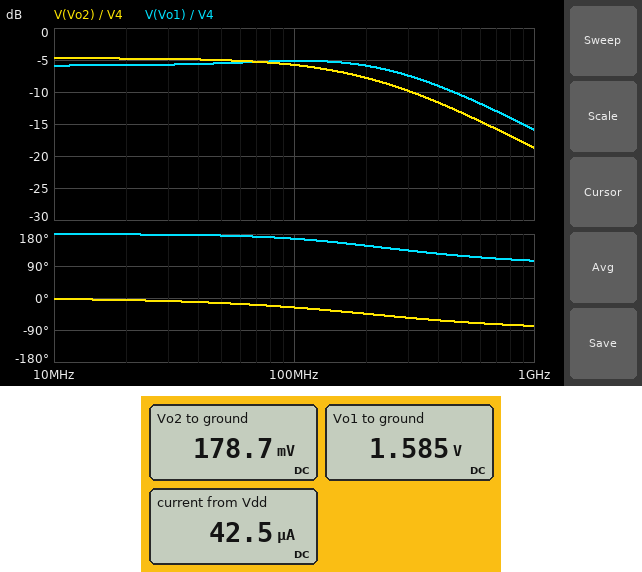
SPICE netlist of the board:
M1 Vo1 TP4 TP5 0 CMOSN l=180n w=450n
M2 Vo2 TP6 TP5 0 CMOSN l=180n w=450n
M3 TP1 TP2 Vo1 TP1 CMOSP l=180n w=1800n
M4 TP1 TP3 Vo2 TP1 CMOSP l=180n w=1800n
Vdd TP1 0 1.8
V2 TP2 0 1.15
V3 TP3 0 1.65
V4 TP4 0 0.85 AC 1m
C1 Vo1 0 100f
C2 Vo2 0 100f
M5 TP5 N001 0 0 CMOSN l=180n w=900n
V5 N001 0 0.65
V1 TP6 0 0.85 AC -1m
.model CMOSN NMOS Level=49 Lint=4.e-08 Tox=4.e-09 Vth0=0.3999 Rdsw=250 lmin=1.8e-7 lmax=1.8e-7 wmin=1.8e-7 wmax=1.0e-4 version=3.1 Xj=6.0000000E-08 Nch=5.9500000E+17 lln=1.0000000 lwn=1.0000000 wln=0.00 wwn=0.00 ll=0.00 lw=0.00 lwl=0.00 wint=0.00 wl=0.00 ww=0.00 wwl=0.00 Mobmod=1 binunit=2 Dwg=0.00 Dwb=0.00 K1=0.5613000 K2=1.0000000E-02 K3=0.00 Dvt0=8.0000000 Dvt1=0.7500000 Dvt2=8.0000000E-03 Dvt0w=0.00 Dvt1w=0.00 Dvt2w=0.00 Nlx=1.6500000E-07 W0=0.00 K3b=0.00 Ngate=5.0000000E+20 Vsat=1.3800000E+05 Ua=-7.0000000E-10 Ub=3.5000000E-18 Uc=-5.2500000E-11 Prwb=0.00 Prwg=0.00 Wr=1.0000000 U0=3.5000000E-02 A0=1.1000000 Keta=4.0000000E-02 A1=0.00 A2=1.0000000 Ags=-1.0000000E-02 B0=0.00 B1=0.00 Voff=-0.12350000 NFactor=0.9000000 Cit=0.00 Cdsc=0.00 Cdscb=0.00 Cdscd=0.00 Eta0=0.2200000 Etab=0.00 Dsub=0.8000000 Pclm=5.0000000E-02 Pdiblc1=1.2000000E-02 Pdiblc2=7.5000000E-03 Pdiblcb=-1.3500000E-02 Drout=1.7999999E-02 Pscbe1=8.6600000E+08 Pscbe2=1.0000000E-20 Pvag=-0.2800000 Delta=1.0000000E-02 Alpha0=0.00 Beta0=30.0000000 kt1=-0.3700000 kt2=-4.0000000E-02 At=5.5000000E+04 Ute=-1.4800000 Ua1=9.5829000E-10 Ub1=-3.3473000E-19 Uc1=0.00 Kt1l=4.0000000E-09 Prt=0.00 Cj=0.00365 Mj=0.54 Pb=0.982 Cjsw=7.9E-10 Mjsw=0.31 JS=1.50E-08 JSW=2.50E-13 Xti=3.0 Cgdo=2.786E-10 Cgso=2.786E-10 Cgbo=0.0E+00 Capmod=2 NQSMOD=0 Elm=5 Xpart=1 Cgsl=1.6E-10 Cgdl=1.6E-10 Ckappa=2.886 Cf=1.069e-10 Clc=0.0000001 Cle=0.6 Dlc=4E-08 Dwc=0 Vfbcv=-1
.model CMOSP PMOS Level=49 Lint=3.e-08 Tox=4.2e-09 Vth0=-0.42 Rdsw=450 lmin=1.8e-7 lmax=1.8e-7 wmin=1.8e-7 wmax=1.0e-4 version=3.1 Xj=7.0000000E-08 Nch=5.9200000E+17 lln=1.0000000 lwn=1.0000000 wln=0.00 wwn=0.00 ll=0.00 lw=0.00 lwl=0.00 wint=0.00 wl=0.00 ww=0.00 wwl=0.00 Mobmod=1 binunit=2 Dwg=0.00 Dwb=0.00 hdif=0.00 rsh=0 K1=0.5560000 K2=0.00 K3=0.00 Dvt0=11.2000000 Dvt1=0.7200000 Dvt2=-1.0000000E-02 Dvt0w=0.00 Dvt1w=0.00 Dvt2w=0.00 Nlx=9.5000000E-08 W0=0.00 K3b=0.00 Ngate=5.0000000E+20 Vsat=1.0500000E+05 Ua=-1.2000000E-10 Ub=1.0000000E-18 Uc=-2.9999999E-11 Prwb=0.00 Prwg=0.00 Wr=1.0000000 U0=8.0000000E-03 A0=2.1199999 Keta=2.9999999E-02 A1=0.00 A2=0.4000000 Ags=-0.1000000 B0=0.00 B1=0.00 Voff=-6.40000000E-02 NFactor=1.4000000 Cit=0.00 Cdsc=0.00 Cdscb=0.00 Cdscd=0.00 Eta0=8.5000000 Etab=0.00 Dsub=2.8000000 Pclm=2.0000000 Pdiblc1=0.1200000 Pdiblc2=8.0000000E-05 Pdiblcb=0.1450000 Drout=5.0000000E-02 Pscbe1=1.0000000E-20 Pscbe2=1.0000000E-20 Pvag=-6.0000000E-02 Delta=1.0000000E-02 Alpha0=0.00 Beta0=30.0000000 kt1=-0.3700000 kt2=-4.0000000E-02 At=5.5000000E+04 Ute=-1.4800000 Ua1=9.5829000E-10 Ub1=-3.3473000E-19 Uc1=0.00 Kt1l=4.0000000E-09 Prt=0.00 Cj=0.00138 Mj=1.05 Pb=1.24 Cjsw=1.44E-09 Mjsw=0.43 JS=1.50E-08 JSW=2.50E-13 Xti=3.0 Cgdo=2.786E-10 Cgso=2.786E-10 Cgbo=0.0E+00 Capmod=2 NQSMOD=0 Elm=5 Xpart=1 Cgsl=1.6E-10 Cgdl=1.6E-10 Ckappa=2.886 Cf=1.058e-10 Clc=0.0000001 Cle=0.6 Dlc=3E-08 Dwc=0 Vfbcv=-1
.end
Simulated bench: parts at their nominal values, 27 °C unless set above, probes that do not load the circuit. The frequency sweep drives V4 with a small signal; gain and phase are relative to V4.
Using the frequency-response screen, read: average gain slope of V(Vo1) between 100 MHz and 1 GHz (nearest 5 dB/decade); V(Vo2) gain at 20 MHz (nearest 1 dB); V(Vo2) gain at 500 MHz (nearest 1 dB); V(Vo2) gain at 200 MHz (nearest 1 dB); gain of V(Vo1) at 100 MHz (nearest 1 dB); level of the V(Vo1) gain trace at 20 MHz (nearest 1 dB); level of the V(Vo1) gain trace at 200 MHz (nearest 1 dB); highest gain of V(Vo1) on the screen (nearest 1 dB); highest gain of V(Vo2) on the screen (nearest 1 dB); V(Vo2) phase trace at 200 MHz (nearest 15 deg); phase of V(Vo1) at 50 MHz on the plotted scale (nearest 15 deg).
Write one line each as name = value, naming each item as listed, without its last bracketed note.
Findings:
average gain slope of V(Vo1) between 100 MHz and 1 GHz = -10 dB/decade
V(Vo2) gain at 20 MHz = -5 dB
V(Vo2) gain at 500 MHz = -13 dB
V(Vo2) gain at 200 MHz = -8 dB
gain of V(Vo1) at 100 MHz = -5 dB
level of the V(Vo1) gain trace at 20 MHz = -6 dB
level of the V(Vo1) gain trace at 200 MHz = -6 dB
highest gain of V(Vo1) on the screen = -5 dB
highest gain of V(Vo2) on the screen = -5 dB
V(Vo2) phase trace at 200 MHz = -45 deg
phase of V(Vo1) at 50 MHz on the plotted scale = 180 deg
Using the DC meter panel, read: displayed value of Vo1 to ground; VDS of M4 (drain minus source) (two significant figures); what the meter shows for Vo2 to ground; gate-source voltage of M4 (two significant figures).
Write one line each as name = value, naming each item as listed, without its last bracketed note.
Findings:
displayed value of Vo1 to ground = 1.585 V
VDS of M4 (drain minus source) = 1.6 V
what the meter shows for Vo2 to ground = 178.7 mV
gate-source voltage of M4 = 1.5 V
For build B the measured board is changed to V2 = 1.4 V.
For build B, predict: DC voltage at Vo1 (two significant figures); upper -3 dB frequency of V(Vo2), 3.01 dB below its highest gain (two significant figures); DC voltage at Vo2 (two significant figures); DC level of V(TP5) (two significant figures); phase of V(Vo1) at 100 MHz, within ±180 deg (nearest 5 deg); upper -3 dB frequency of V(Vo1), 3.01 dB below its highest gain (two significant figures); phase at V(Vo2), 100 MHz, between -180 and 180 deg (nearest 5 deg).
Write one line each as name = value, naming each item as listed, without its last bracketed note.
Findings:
DC voltage at Vo1 = 96 mV
upper -3 dB frequency of V(Vo2), 3.01 dB below its highest gain = 720 MHz
DC voltage at Vo2 = 43 mV
DC level of V(TP5) = 42 mV
phase of V(Vo1) at 100 MHz, within ±180 deg = 155 deg
upper -3 dB frequency of V(Vo1), 3.01 dB below its highest gain = 210 MHz
phase at V(Vo2), 100 MHz, between -180 and 180 deg = 40 deg
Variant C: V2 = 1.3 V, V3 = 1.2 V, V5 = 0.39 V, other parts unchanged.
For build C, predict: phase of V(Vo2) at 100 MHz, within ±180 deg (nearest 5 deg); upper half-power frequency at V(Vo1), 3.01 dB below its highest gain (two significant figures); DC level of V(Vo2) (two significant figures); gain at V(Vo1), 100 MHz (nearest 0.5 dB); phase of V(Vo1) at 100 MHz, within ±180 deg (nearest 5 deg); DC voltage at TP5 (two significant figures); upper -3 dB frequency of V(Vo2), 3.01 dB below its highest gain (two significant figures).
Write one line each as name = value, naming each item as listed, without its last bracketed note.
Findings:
phase of V(Vo2) at 100 MHz, within ±180 deg = -15 deg
upper half-power frequency at V(Vo1), 3.01 dB below its highest gain = 250 MHz
DC level of V(Vo2) = 1.8 V
gain at V(Vo1), 100 MHz = -23.5 dB
phase of V(Vo1) at 100 MHz, within ±180 deg = 160 deg
DC voltage at TP5 = 460 mV
upper -3 dB frequency of V(Vo2), 3.01 dB below its highest gain = 380 MHz
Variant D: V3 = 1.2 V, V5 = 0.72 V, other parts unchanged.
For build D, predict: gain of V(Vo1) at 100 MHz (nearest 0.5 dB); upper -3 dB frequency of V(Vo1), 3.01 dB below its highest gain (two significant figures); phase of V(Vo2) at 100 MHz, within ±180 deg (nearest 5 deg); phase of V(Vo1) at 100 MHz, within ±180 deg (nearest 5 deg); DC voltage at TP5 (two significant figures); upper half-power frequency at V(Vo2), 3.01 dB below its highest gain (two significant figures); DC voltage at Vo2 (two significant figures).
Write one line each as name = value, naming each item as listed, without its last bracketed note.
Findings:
gain of V(Vo1) at 100 MHz = -4.5 dB
upper -3 dB frequency of V(Vo1), 3.01 dB below its highest gain = 270 MHz
phase of V(Vo2) at 100 MHz, within ±180 deg = -35 deg
phase of V(Vo1) at 100 MHz, within ±180 deg = 160 deg
DC voltage at TP5 = 220 mV
upper half-power frequency at V(Vo2), 3.01 dB below its highest gain = 140 MHz
DC voltage at Vo2 = 1.6 V
